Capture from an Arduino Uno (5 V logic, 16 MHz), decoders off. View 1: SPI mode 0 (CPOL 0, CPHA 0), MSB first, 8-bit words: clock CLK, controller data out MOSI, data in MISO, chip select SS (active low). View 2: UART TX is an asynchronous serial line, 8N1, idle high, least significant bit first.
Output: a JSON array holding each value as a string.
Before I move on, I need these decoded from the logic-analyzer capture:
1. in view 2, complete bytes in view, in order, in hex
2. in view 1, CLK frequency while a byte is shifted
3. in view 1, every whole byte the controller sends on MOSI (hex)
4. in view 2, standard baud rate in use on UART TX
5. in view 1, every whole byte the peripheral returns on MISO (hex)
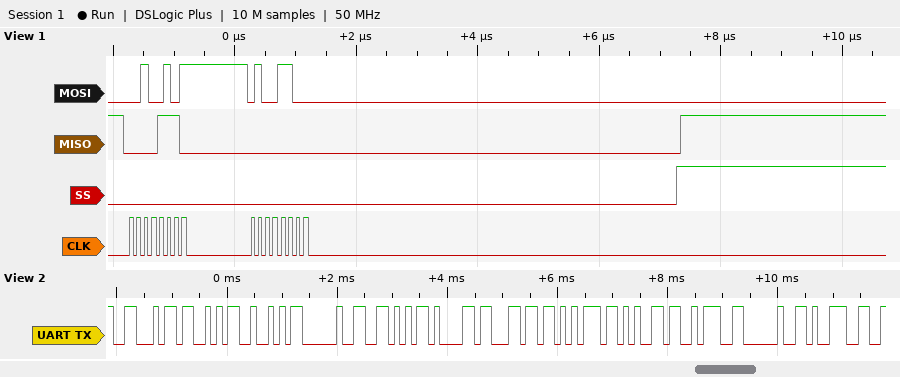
["0x46 0x53 0x52 0x20 0x56 0x61 0x6C 0x75 0x65 0x3A 0x20 0x39", "8 MHz", "0x25 0x4C", "9600 baud", "0x0E 0x00"]
